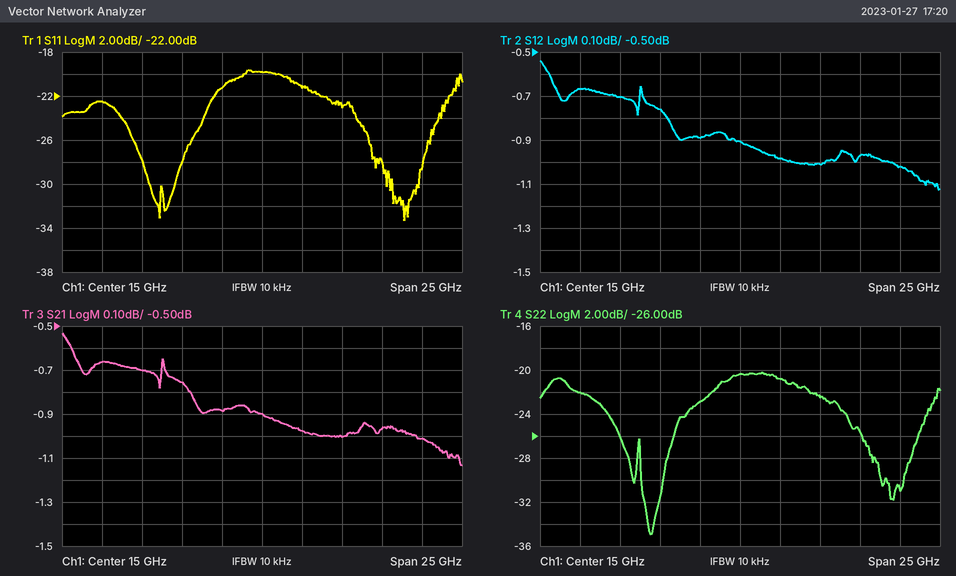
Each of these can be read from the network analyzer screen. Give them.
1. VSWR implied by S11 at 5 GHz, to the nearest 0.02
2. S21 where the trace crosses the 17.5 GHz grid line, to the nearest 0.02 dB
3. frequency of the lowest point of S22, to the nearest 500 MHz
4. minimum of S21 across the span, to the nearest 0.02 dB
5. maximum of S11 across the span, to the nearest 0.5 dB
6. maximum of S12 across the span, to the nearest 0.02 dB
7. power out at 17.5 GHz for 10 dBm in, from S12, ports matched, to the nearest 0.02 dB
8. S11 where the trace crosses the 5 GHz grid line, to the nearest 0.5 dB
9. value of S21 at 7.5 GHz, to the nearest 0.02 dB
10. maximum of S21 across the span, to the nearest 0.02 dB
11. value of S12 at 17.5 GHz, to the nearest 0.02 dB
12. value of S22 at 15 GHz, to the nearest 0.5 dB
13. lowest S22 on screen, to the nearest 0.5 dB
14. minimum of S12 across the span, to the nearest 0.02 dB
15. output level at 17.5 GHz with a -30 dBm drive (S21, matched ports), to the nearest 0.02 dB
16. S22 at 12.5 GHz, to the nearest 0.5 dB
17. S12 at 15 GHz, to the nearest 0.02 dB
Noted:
1.16
-0.98 dB
9.5 GHz
-1.14 dB
-19.5 dB
-0.54 dB
9.02 dBm
-22.5 dB
-0.70 dB
-0.54 dB
-0.98 dB
-20.5 dB
-35.0 dB
-1.12 dB
-30.98 dBm
-23.0 dB
-0.90 dB
